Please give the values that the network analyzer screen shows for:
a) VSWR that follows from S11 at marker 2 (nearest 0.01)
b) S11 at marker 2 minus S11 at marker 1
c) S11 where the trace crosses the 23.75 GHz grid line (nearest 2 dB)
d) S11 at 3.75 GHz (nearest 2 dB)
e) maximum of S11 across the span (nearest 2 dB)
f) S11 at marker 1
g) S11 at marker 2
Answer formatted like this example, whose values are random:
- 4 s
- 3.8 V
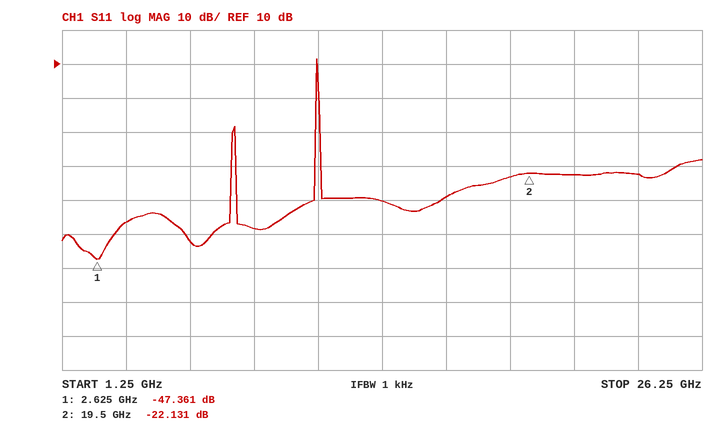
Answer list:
- 1.17
- 25.230 dB
- -22 dB
- -36 dB
- 12 dB
- -47.361 dB
- -22.131 dB
